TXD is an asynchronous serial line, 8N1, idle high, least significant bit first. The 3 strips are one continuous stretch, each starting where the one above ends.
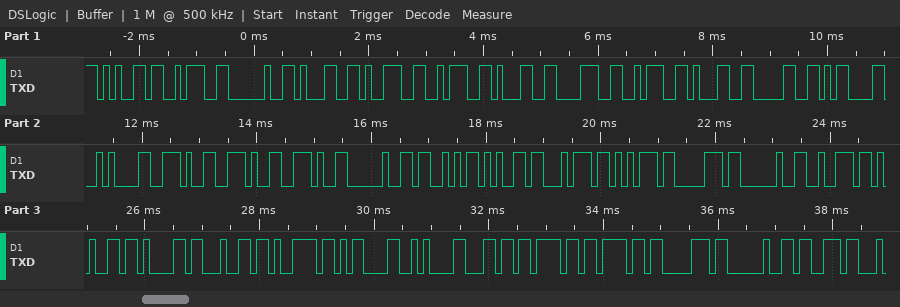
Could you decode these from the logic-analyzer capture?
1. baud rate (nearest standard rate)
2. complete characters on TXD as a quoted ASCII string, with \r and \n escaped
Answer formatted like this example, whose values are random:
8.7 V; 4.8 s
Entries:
9600 baud; "e: 19:18:10\r\n... Setup ready\r\nloop s"
